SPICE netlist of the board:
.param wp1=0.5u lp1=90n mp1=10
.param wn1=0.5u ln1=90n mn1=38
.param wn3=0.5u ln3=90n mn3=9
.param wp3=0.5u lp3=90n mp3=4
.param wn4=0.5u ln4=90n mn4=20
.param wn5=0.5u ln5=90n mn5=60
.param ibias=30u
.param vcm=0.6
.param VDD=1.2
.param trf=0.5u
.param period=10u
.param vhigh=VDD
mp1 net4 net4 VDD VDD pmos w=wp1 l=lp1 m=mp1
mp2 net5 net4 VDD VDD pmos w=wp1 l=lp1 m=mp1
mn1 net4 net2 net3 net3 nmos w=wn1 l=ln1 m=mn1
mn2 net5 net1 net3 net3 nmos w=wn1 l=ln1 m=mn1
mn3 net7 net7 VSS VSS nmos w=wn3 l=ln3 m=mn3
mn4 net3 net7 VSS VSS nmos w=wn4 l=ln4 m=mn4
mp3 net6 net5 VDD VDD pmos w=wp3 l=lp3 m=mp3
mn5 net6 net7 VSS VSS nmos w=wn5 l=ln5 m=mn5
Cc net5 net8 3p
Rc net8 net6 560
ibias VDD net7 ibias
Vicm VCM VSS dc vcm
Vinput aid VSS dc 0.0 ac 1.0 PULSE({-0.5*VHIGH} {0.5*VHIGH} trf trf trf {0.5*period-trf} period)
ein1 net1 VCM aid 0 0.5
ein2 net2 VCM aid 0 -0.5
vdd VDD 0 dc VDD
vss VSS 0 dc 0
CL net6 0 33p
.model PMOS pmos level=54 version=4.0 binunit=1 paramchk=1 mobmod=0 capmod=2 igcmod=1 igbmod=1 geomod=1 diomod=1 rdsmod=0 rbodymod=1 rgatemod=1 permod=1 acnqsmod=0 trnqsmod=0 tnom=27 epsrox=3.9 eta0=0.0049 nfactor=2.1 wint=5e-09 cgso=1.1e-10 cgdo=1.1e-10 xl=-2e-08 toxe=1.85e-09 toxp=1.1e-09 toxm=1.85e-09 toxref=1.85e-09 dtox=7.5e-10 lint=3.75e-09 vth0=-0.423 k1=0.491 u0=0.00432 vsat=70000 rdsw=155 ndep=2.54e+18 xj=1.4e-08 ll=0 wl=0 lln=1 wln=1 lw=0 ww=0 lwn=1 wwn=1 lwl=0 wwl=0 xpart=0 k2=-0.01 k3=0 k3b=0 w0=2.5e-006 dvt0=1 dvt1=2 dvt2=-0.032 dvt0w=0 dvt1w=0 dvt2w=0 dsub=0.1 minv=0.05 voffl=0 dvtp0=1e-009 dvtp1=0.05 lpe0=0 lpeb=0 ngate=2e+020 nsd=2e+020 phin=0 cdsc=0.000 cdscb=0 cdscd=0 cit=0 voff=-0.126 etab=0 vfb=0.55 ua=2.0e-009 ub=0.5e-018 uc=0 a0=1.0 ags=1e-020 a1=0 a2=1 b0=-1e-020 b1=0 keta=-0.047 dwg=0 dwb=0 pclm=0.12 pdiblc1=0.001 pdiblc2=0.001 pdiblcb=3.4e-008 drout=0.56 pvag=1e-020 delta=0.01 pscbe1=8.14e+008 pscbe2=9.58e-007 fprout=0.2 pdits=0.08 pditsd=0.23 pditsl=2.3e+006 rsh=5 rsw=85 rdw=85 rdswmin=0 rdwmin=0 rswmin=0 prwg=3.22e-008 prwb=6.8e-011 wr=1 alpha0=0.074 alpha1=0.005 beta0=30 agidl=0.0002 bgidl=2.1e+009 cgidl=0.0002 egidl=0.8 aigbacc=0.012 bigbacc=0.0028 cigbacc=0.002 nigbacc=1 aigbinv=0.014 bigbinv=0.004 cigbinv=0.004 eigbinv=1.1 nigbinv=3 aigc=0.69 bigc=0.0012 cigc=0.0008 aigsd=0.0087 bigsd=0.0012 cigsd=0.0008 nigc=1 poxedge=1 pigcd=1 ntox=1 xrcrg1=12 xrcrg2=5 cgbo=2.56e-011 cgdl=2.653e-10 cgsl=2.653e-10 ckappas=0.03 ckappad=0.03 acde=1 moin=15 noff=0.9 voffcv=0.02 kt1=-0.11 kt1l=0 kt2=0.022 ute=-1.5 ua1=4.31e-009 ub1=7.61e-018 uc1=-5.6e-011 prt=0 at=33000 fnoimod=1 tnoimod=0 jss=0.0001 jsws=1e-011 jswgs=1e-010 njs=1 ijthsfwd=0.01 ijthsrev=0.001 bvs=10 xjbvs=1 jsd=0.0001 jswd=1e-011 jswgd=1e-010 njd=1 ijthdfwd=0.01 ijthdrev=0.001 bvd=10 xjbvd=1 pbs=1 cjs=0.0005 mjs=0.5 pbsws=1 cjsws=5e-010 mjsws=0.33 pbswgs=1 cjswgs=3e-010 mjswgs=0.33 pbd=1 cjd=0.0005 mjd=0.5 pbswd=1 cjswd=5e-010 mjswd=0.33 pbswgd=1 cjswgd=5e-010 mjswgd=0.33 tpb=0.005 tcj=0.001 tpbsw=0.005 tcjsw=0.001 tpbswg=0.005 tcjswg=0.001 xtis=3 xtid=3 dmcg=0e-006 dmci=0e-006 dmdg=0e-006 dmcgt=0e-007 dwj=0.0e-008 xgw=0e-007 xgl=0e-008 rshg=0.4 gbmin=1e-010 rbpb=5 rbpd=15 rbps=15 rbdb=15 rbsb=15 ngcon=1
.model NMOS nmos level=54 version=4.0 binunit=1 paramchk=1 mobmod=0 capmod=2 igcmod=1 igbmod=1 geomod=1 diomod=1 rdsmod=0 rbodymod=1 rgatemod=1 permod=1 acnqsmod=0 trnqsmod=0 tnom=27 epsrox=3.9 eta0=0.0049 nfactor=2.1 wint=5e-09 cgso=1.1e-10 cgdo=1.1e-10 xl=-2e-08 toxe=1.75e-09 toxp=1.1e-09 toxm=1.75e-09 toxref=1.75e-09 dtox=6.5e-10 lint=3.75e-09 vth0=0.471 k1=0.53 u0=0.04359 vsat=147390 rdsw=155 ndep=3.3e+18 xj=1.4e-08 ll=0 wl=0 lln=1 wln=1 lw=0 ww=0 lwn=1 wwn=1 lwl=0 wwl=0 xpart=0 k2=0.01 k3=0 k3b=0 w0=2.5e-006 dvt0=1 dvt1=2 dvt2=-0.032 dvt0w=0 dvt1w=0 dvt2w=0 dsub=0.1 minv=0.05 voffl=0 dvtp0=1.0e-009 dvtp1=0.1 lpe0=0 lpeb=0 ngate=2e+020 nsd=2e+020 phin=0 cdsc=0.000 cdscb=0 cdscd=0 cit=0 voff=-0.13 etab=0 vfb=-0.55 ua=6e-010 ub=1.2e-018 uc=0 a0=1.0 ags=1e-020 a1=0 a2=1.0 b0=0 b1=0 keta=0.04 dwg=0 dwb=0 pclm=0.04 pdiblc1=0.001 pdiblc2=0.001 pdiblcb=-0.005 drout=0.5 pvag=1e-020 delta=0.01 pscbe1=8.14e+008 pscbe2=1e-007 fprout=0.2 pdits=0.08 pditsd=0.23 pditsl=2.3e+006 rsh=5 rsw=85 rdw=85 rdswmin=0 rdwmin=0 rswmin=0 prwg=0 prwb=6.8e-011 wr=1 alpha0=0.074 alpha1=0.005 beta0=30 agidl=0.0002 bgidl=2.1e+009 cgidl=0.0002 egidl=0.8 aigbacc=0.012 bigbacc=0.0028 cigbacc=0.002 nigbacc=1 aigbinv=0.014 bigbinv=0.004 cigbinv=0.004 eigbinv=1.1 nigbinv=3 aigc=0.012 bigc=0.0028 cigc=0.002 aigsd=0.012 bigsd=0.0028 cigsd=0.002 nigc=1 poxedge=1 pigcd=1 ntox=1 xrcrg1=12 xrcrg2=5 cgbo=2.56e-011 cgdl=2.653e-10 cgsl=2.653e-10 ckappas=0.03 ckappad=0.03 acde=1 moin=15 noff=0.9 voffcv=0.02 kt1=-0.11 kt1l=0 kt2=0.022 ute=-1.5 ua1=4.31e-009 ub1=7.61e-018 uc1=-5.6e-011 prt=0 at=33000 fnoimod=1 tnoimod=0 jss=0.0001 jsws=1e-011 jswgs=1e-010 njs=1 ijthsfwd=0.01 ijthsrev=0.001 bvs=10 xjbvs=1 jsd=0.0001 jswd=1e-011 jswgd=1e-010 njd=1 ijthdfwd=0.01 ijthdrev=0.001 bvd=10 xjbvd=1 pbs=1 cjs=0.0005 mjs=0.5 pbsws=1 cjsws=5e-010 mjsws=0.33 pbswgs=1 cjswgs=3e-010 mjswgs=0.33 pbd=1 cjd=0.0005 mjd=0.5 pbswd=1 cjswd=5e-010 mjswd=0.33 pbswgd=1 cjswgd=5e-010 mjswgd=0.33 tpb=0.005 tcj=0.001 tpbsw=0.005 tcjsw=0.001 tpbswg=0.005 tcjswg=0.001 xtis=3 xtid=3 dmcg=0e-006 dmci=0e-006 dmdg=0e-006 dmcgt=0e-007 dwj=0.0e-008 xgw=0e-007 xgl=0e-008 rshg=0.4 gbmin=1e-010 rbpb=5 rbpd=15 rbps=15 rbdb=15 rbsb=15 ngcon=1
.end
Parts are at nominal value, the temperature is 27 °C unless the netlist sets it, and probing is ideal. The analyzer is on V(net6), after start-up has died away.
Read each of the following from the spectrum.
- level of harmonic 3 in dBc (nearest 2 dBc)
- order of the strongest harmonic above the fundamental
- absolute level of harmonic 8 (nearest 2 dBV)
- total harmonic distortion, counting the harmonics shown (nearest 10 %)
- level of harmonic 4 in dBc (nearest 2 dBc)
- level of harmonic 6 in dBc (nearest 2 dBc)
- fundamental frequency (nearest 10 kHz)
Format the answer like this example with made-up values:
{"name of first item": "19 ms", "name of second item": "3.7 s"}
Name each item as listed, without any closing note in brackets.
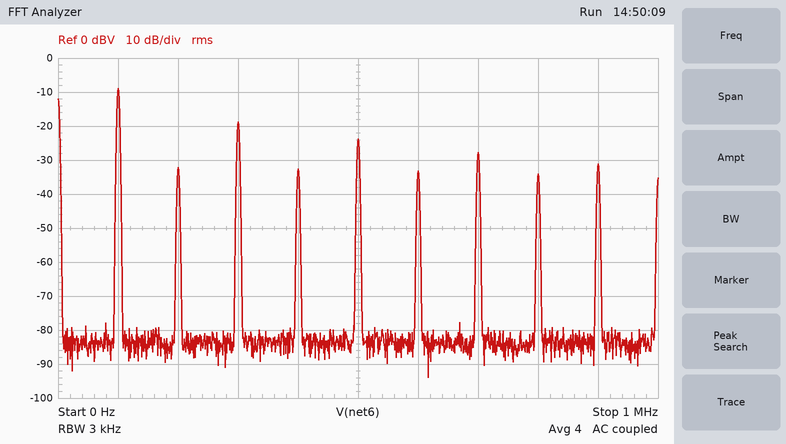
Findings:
{"level of harmonic 3 in dBc": "-10 dBc", "order of the strongest harmonic above the fundamental": "3", "absolute level of harmonic 8": "-34 dBV", "total harmonic distortion, counting the harmonics shown": "40 %", "level of harmonic 4 in dBc": "-24 dBc", "level of harmonic 6 in dBc": "-24 dBc", "fundamental frequency": "100 kHz"}
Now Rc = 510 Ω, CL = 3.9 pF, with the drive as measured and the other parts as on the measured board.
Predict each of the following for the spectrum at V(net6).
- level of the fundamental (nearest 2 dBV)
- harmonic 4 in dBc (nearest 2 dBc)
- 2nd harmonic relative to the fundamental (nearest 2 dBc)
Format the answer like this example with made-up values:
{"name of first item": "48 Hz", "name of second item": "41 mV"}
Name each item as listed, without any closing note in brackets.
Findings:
{"level of the fundamental": "-8 dBV", "harmonic 4 in dBc": "-26 dBc", "2nd harmonic relative to the fundamental": "-26 dBc"}
